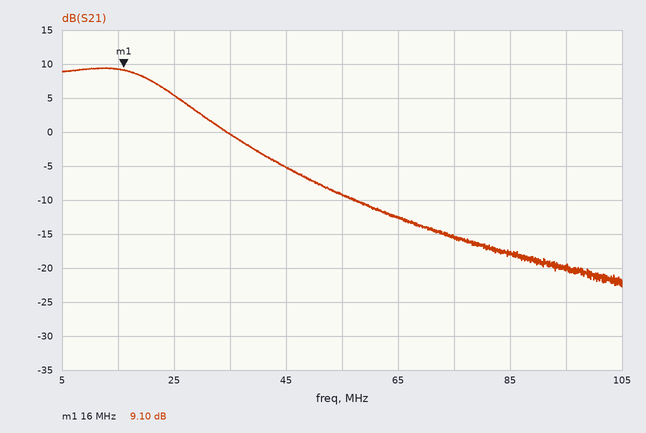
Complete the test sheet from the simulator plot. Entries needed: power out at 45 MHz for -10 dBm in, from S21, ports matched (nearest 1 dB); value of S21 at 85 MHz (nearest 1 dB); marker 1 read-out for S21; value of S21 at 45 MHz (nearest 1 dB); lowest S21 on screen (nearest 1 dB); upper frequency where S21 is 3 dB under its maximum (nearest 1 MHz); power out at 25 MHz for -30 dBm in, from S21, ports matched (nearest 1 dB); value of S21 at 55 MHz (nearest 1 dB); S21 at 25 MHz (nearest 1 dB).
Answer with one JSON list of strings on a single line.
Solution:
["-15 dBm", "-18 dB", "9.10 dB", "-5 dB", "-23 dB", "23 MHz", "-25 dBm", "-9 dB", "5 dB"]
